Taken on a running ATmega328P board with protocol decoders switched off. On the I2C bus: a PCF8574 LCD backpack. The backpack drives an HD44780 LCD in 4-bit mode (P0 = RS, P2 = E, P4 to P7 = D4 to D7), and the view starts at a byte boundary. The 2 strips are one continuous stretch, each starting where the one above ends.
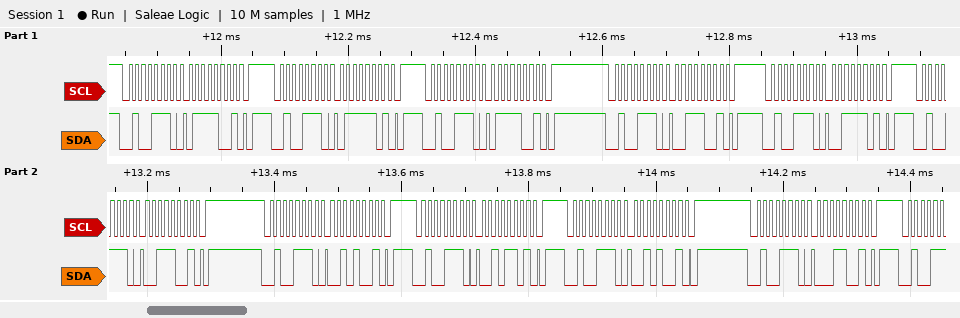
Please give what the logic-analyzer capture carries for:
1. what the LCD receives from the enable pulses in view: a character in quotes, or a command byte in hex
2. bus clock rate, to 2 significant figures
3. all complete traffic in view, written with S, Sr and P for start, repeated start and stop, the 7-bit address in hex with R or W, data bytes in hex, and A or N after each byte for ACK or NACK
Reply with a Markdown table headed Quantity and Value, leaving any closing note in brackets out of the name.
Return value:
| Quantity | Value |
|---|---|
| what the LCD receives from the enable pulses in view: a character in quotes, or a command byte in hex | 's' |
| bus clock rate, to 2 significant figures | 100 kHz |
| all complete traffic in view, written with S, Sr and P for start, repeated start and stop, the 7-bit address in hex with R or W, data bytes in hex, and A or N after each byte for ACK or NACK | S 27W A 79 A P S 27W A 7D A P S 27W A 79 A P S 27W A 39 A P S 27W A 3D A P S 27W A 39 A P S 27W A 29 A P S 27W A 2D A P S 27W A 29 A P S 27W A 19 A P |
